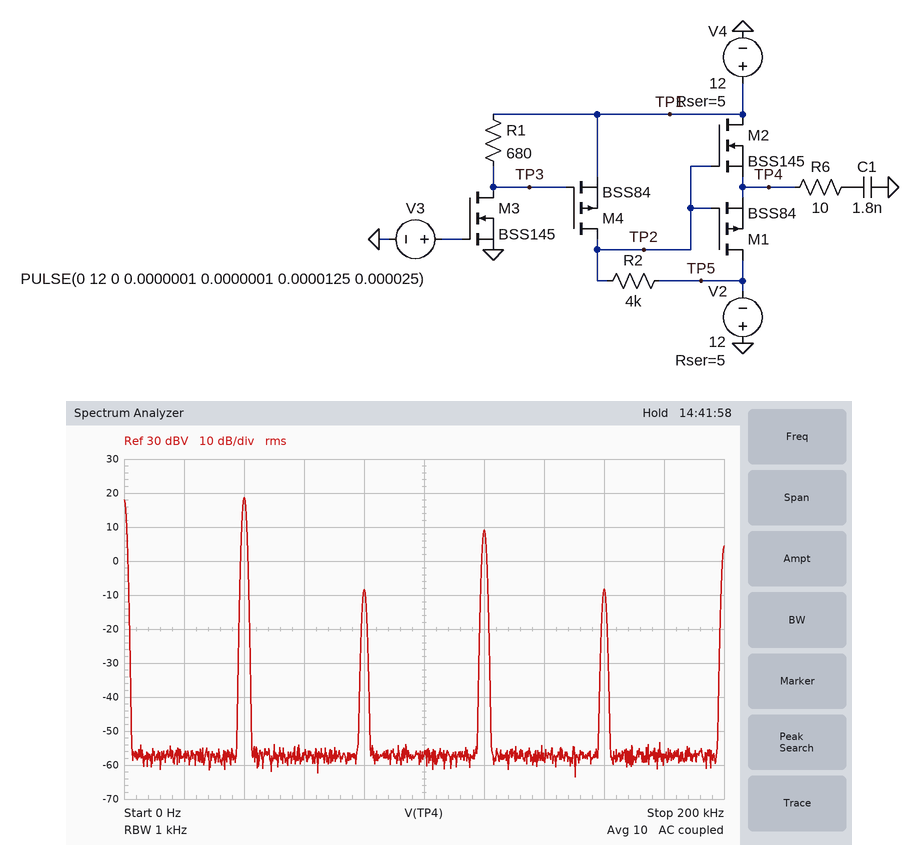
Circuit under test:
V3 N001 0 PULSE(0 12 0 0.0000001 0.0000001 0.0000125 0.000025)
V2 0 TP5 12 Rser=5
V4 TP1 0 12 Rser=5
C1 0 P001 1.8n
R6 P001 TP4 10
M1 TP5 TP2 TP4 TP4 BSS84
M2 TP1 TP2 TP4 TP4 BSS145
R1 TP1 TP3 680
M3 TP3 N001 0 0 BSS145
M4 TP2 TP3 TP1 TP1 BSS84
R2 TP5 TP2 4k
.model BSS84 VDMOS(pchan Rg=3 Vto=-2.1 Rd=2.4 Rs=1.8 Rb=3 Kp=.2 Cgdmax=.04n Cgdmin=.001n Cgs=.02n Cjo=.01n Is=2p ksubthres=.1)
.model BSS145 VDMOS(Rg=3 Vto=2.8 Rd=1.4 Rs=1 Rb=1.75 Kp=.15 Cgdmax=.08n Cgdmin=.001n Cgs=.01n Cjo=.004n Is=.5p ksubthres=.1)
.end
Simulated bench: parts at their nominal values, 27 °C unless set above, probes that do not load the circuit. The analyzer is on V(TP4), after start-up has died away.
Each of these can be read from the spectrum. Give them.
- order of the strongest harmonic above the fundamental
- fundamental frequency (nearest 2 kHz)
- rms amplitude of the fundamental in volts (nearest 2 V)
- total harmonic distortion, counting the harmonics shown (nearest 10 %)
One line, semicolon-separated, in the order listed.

3; 40 kHz; 8 V; 30 %
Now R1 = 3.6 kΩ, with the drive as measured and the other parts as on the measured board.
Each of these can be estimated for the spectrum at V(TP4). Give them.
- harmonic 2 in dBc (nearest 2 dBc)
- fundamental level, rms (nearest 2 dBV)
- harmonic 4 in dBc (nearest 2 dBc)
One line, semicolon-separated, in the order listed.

-20 dBc; 18 dBV; -20 dBc
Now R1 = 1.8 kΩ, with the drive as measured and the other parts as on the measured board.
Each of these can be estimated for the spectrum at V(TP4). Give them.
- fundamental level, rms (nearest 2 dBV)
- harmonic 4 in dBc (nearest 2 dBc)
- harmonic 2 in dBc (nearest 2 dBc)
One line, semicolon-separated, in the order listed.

18 dBV; -24 dBc; -24 dBc
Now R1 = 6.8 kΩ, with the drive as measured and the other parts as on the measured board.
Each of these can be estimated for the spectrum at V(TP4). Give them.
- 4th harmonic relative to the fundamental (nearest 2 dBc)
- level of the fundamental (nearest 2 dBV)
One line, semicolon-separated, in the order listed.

-16 dBc; 18 dBV
